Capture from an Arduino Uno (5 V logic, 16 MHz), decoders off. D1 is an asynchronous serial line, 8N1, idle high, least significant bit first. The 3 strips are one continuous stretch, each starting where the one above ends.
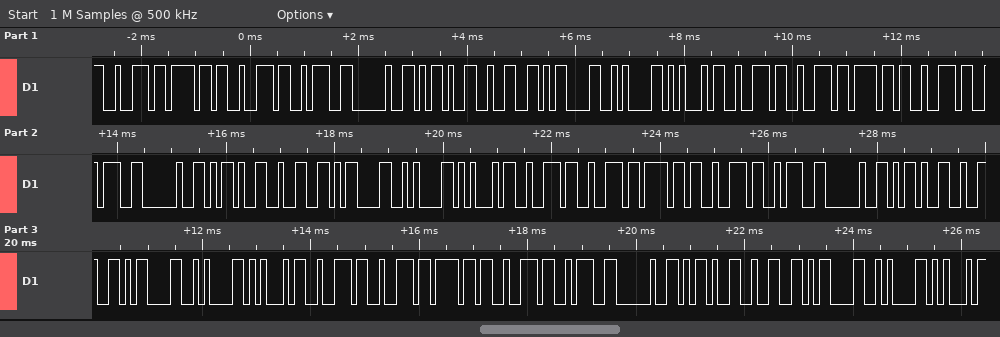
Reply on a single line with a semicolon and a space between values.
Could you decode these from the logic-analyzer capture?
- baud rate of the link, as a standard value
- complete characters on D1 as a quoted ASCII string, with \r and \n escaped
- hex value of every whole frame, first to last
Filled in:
9600 baud; "ror: -2\r\nError: -2\r\nError: -2\r\nError: -2\r\nE"; 0x72 0x6F 0x72 0x3A 0x20 0x2D 0x32 0x0D 0x0A 0x45 0x72 0x72 0x6F 0x72 0x3A 0x20 0x2D 0x32 0x0D 0x0A 0x45 0x72 0x72 0x6F 0x72 0x3A 0x20 0x2D 0x32 0x0D 0x0A 0x45 0x72 0x72 0x6F 0x72 0x3A 0x20 0x2D 0x32 0x0D 0x0A 0x45
